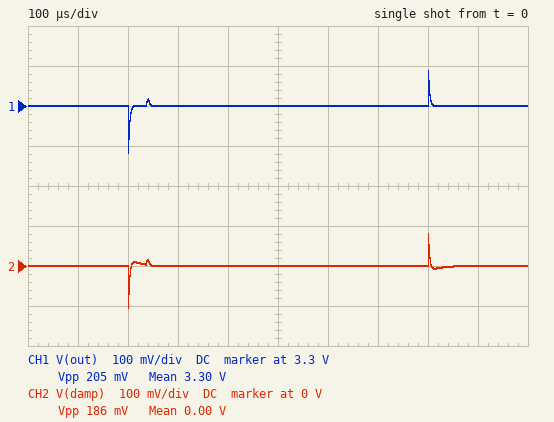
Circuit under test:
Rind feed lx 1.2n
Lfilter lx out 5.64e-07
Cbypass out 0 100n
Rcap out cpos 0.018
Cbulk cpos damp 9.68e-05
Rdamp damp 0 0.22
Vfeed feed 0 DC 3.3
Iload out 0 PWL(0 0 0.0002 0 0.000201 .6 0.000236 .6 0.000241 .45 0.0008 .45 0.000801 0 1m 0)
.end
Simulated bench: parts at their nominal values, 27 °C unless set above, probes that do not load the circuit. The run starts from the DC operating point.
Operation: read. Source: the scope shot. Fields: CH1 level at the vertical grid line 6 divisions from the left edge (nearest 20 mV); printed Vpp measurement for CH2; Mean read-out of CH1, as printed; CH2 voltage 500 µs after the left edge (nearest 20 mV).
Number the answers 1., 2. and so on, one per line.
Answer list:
1. 3.30 V
2. 186 mV
3. 3.30 V
4. 0 V
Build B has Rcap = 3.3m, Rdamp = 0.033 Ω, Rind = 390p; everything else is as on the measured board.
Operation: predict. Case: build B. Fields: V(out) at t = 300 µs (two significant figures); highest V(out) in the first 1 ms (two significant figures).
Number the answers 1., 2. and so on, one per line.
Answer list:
1. 3.3 V
2. 3.3 V
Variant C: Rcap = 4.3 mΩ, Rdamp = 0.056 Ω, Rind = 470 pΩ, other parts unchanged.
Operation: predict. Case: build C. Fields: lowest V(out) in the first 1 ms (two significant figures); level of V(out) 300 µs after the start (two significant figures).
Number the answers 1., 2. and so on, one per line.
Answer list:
1. 3.3 V
2. 3.3 V
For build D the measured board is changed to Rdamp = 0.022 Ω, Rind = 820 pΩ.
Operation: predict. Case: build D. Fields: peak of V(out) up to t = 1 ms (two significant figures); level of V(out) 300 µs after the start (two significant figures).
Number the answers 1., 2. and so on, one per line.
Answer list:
1. 3.3 V
2. 3.3 V
